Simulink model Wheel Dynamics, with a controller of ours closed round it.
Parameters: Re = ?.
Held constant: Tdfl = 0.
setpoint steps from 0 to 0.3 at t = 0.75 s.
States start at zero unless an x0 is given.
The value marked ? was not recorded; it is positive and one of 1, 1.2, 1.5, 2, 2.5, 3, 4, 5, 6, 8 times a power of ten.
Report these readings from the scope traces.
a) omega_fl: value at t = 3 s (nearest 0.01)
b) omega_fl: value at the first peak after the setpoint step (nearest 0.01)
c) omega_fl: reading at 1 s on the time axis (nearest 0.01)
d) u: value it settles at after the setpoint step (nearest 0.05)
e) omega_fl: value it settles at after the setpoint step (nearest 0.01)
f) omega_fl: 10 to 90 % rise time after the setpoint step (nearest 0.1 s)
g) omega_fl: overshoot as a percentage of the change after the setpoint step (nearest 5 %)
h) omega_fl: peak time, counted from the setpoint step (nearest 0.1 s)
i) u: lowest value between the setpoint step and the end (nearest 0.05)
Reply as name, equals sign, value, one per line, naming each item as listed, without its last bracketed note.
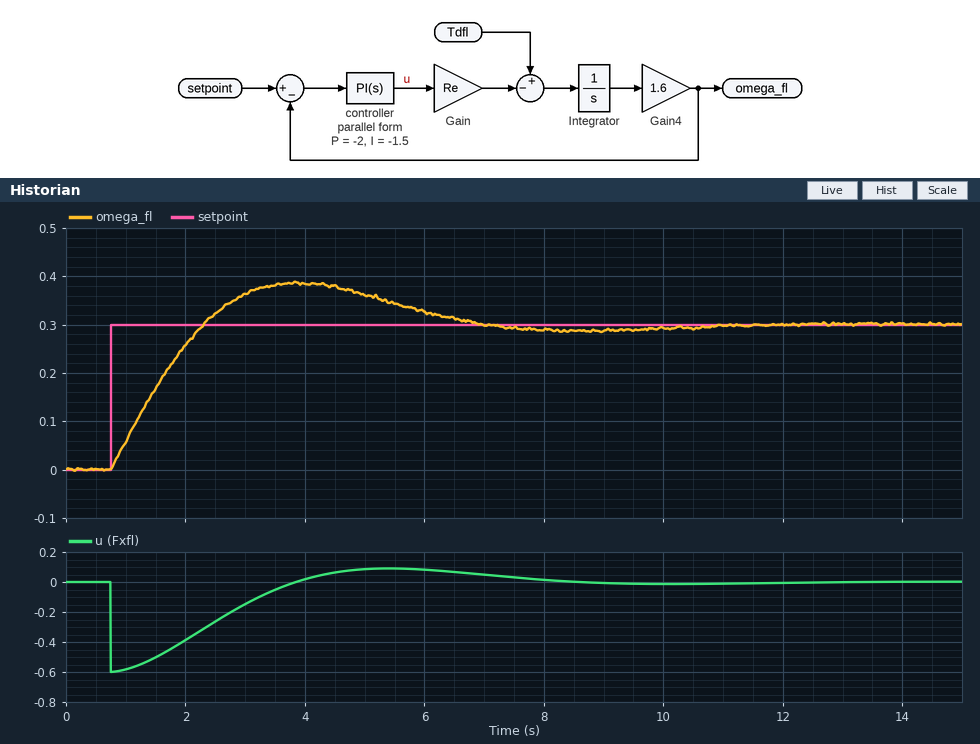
omega_fl: value at t = 3 s = 0.36
omega_fl: value at the first peak after the setpoint step = 0.39
omega_fl: reading at 1 s on the time axis = 0.06
u: value it settles at after the setpoint step = 0.00
omega_fl: value it settles at after the setpoint step = 0.30
omega_fl: 10 to 90 % rise time after the setpoint step = 1.2 s
omega_fl: overshoot as a percentage of the change after the setpoint step = 30 %
omega_fl: peak time, counted from the setpoint step = 3.1 s
u: lowest value between the setpoint step and the end = -0.60
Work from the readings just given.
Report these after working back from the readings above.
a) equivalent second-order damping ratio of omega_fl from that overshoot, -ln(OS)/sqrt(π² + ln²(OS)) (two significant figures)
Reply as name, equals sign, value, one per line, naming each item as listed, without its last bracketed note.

equivalent second-order damping ratio of omega_fl from that overshoot, -ln(OS)/sqrt(π² + ln²(OS)) = 0.36
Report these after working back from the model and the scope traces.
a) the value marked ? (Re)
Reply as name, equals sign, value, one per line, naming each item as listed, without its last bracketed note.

the value marked ? = 0.25
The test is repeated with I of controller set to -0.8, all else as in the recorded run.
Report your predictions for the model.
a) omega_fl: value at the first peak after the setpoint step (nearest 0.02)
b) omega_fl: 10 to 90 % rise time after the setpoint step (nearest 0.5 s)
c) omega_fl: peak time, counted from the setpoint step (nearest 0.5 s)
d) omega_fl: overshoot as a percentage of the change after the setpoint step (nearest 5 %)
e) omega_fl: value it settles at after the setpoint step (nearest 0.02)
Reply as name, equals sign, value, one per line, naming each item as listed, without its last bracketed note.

omega_fl: value at the first peak after the setpoint step = 0.36
omega_fl: 10 to 90 % rise time after the setpoint step = 1.5 s
omega_fl: peak time, counted from the setpoint step = 4.0 s
omega_fl: overshoot as a percentage of the change after the setpoint step = 20 %
omega_fl: value it settles at after the setpoint step = 0.30
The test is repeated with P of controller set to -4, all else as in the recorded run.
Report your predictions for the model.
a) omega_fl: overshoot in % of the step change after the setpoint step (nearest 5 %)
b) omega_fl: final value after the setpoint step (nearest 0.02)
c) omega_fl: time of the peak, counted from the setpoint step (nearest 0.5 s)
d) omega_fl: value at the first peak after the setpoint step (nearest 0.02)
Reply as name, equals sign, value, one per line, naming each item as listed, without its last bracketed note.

omega_fl: overshoot in % of the step change after the setpoint step = 15 %
omega_fl: final value after the setpoint step = 0.30
omega_fl: time of the peak, counted from the setpoint step = 2.5 s
omega_fl: value at the first peak after the setpoint step = 0.34
